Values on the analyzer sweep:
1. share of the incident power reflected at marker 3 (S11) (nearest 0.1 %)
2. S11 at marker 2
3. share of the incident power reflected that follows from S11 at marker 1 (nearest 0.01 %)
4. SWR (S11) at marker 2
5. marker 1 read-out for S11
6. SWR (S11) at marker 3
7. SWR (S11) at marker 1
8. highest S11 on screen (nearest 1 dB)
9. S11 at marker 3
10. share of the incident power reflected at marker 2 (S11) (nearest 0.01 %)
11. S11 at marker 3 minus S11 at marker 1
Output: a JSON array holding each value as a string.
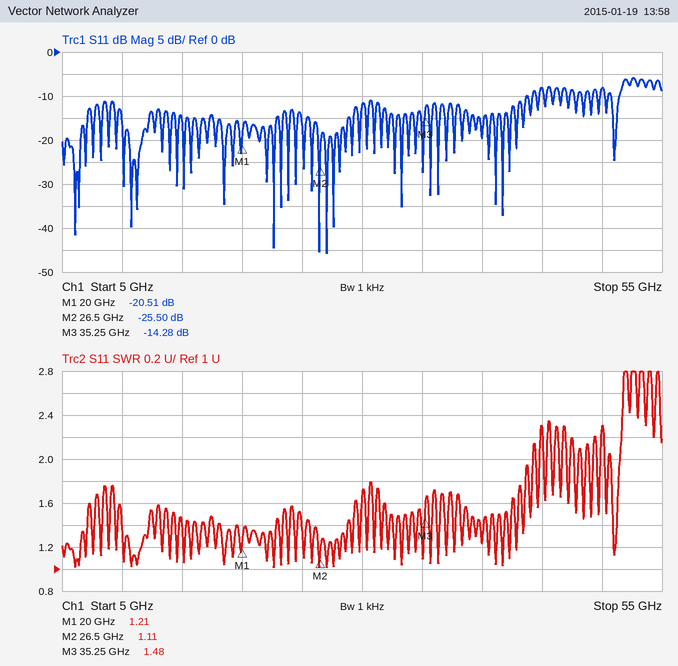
["3.7 %", "-25.50 dB", "0.89 %", "1.11", "-20.51 dB", "1.48", "1.21", "-6 dB", "-14.28 dB", "0.28 %", "6.23 dB"]
